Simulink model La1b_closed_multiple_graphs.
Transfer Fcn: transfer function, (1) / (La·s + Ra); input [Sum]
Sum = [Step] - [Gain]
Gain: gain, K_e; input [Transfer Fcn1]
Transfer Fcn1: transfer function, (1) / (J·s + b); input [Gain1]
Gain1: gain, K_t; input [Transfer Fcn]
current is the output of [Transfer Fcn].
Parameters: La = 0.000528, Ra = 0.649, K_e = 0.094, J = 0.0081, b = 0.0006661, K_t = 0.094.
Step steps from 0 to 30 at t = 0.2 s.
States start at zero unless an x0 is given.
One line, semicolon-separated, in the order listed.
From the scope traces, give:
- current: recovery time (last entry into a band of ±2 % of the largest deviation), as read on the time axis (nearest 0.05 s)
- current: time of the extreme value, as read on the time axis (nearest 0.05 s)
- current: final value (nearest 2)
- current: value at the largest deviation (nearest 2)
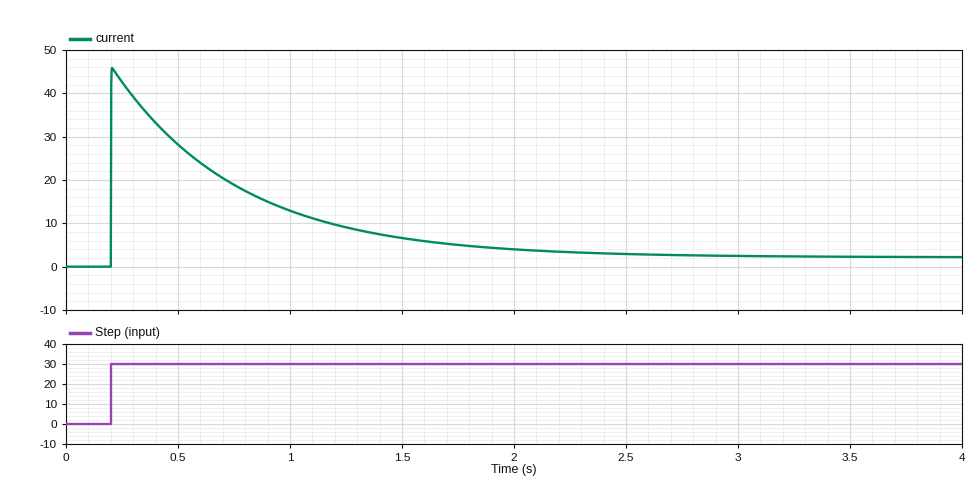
2.40 s; 0.20 s; 2; 46
